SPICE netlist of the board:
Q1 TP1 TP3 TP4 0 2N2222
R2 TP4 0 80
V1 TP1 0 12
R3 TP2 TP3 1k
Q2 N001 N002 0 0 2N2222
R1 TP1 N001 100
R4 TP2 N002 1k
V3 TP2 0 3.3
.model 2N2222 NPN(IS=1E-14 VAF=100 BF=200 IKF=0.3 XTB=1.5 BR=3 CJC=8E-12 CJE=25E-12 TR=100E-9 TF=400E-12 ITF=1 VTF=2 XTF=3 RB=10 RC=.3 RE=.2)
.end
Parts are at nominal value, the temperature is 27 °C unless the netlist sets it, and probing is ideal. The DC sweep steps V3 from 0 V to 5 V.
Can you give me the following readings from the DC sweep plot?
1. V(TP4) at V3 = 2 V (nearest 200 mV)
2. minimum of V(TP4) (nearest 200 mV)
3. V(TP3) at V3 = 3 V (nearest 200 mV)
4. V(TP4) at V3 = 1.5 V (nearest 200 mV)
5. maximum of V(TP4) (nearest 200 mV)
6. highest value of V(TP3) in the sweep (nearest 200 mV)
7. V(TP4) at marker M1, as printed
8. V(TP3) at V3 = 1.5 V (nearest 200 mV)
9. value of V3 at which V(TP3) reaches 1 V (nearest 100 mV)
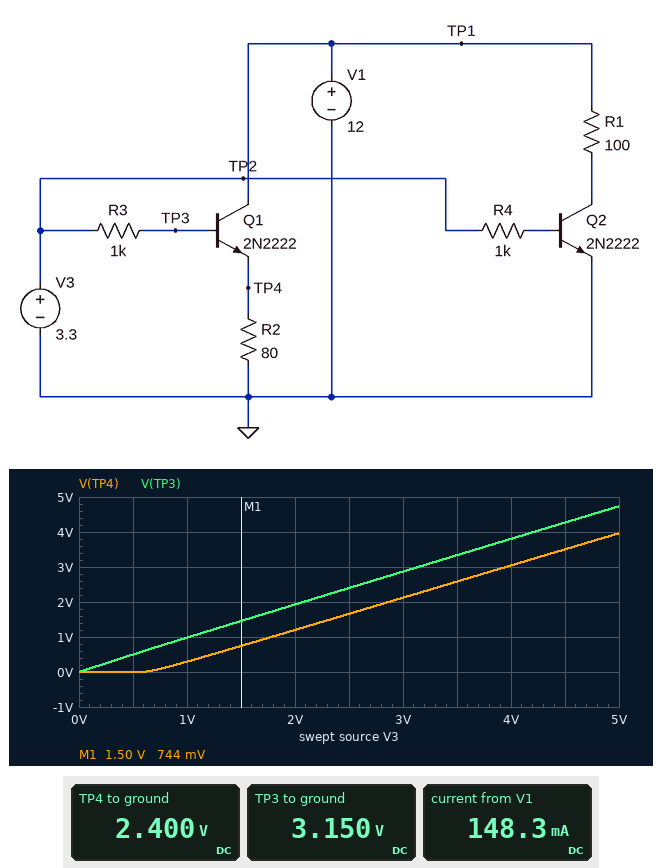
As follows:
1.2 V
0 V
2.8 V
800 mV
4.0 V
4.8 V
744 mV
1.4 V
1.0 V
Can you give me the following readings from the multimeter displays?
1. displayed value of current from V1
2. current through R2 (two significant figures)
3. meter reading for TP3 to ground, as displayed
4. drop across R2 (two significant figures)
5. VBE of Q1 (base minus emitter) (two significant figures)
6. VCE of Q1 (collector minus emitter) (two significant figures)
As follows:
148.3 mA
30 mA
3.150 V
2.4 V
750 mV
9.6 V
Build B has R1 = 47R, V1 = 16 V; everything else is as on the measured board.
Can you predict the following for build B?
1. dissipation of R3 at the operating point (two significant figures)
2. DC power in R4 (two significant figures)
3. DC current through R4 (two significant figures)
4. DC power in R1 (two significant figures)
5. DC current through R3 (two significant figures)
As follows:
21 µW
5.8 mW
2.4 mA
3.3 W
140 µA
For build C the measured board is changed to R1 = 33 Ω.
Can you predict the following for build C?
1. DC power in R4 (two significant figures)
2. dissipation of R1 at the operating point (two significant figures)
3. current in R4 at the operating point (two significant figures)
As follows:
5.8 mW
2.3 W
2.4 mA
